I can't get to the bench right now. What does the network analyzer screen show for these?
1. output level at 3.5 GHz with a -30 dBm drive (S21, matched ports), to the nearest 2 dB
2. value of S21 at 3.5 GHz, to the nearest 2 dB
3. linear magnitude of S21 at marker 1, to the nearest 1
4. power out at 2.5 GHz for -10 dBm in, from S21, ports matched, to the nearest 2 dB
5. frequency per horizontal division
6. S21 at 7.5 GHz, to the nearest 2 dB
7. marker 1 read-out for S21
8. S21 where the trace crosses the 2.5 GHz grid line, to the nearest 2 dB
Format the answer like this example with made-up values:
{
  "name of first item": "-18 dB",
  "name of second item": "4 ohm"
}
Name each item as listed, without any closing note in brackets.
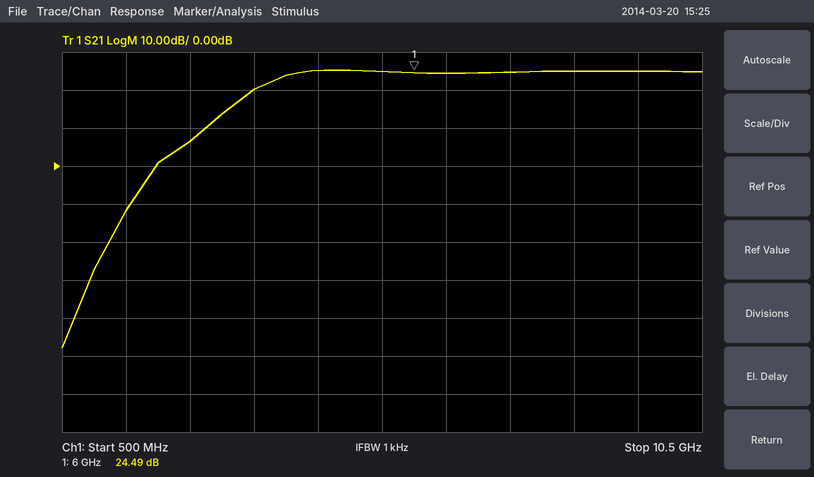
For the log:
{
  "output level at 3.5 GHz with a -30 dBm drive (S21, matched ports), to the nearest 2 dB": "-10 dBm",
  "value of S21 at 3.5 GHz, to the nearest 2 dB": "20 dB",
  "linear magnitude of S21 at marker 1, to the nearest 1": "17",
  "power out at 2.5 GHz for -10 dBm in, from S21, ports matched, to the nearest 2 dB": "-4 dBm",
  "frequency per horizontal division": "1 GHz",
  "S21 at 7.5 GHz, to the nearest 2 dB": "24 dB",
  "marker 1 read-out for S21": "24.49 dB",
  "S21 where the trace crosses the 2.5 GHz grid line, to the nearest 2 dB": "6 dB"
}
